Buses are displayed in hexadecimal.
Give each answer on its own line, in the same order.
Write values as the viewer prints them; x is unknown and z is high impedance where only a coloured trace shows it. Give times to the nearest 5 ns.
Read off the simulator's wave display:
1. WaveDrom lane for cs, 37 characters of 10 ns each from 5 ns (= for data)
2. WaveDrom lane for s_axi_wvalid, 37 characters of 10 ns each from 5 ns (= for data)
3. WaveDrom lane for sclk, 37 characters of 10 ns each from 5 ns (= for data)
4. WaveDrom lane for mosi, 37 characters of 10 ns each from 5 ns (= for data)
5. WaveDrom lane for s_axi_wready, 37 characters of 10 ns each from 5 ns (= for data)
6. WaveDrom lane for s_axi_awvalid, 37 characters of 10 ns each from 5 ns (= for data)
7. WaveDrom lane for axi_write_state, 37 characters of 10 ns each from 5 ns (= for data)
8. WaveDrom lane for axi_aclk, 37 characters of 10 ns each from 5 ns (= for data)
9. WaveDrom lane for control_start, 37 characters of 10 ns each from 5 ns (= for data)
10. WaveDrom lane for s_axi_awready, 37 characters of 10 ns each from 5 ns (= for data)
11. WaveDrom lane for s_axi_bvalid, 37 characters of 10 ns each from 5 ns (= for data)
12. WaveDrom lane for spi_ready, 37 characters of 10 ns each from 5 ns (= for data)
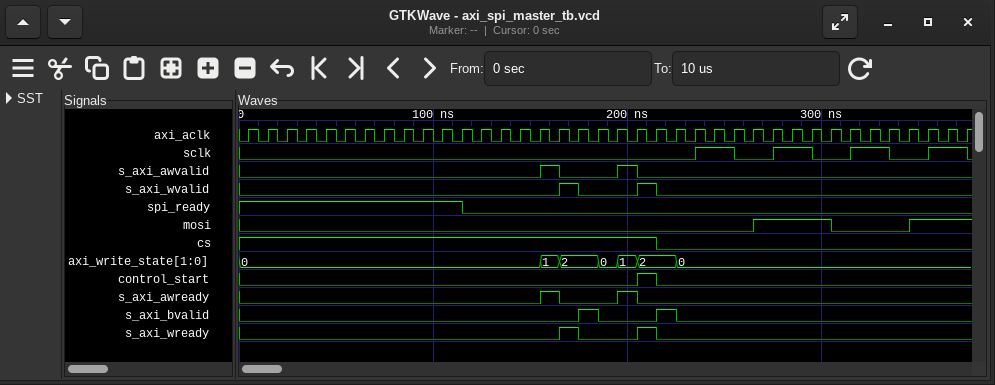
{name: 'cs', wave: '1....................0...............'}
{name: 's_axi_wvalid', wave: '0...............10..10...............'}
{name: 'sclk', wave: '0......................1.0.1.0.1.0.1.'}
{name: 'mosi', wave: '0.........................1...0...1..'}
{name: 's_axi_wready', wave: '0...............10..10...............'}
{name: 's_axi_awvalid', wave: '0..............10..10................'}
{name: 'axi_write_state', wave: '=..............==.===.=..............', data: '0 1 2 0 1 2 0'}
{name: 'axi_aclk', wave: 'p....................................'}
{name: 'control_start', wave: '0...................10...............'}
{name: 's_axi_awready', wave: '0..............10..10................'}
{name: 's_axi_bvalid', wave: '0................10..10..............'}
{name: 'spi_ready', wave: '1..........0.........................'}
